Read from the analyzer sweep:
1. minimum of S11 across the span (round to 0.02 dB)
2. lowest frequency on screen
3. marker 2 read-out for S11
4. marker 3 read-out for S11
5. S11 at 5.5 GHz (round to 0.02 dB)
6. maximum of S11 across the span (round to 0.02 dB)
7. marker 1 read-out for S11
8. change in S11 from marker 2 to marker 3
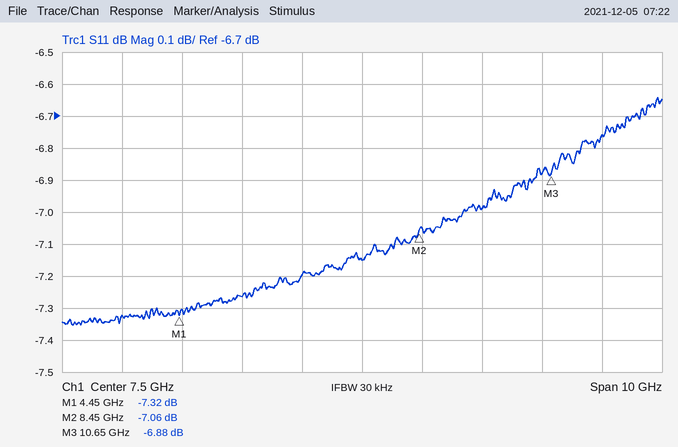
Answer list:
-7.36 dB
2.5 GHz
-7.06 dB
-6.88 dB
-7.26 dB
-6.64 dB
-7.32 dB
0.18 dB
